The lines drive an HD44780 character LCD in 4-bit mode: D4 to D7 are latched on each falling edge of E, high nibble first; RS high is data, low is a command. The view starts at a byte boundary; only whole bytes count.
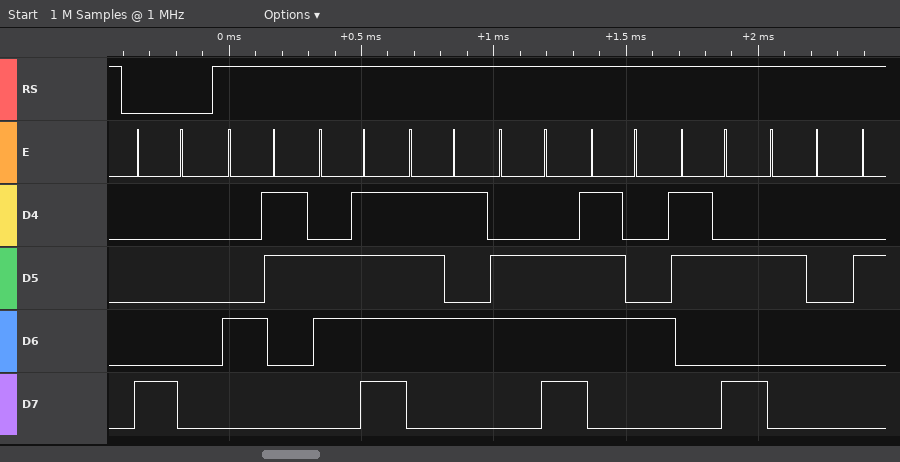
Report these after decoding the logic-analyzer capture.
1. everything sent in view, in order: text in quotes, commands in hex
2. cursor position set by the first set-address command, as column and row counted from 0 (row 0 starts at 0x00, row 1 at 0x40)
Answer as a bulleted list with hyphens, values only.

- 0x80 "Count: "
- column 0, row 0
